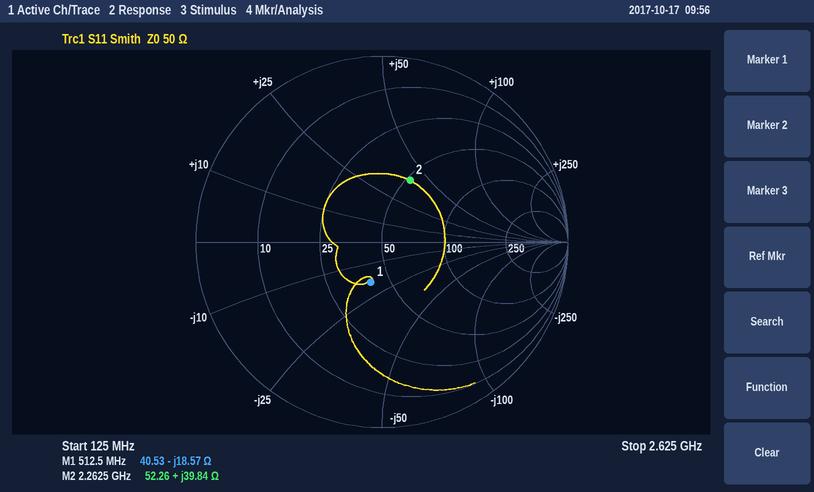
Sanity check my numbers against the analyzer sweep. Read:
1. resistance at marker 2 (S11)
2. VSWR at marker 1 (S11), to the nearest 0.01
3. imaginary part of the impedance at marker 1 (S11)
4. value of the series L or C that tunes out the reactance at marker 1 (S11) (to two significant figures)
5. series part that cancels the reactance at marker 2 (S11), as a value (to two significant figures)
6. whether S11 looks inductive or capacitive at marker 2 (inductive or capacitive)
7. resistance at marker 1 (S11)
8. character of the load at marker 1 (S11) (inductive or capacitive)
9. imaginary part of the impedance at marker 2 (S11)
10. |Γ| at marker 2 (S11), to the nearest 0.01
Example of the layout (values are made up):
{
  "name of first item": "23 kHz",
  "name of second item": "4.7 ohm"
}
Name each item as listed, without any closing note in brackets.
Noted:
{
  "resistance at marker 2": "52.26 Ω",
  "VSWR at marker 1 (S11), to the nearest 0.01": "1.58",
  "imaginary part of the impedance at marker 1": "-18.57 Ω",
  "value of the series L or C that tunes out the reactance at marker 1 (S11)": "5.8 nH",
  "series part that cancels the reactance at marker 2 (S11), as a value": "1.8 pF",
  "whether S11 looks inductive or capacitive at marker 2": "inductive",
  "resistance at marker 1": "40.53 Ω",
  "character of the load at marker 1 (S11)": "capacitive",
  "imaginary part of the impedance at marker 2": "+39.84 Ω",
  "|Γ| at marker 2 (S11), to the nearest 0.01": "0.36"
}
